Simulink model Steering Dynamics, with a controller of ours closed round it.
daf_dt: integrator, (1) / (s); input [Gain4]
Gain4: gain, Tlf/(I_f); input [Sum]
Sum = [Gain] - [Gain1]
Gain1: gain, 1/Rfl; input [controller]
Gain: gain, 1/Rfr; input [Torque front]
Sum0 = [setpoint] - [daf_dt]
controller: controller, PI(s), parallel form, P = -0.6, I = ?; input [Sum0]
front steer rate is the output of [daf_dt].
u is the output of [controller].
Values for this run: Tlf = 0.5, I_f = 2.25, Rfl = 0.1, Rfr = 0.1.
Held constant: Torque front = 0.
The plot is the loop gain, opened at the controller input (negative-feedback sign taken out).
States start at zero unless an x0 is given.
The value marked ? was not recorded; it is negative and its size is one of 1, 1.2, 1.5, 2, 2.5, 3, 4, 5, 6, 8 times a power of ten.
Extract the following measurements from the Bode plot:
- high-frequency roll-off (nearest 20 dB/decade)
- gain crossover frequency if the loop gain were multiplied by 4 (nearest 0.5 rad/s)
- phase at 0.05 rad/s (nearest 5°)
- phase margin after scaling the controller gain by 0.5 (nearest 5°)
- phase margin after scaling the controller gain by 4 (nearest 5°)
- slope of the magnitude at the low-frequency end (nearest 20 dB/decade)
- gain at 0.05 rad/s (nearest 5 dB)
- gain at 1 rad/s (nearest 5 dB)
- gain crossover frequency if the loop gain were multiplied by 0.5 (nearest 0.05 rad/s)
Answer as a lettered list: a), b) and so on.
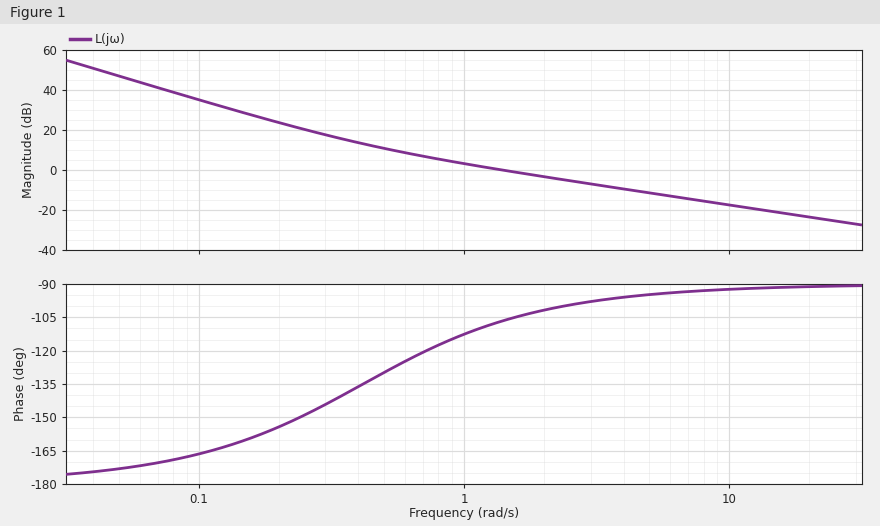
a) -20 dB/decade
b) 5.5 rad/s
c) -175°
d) 60°
e) 85°
f) -40 dB/decade
g) 45 dB
h) 5 dB
i) 0.75 rad/s
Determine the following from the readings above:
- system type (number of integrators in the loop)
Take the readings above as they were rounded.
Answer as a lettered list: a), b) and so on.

a) 2
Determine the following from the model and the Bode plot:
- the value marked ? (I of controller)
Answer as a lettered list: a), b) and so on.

a) -0.25
